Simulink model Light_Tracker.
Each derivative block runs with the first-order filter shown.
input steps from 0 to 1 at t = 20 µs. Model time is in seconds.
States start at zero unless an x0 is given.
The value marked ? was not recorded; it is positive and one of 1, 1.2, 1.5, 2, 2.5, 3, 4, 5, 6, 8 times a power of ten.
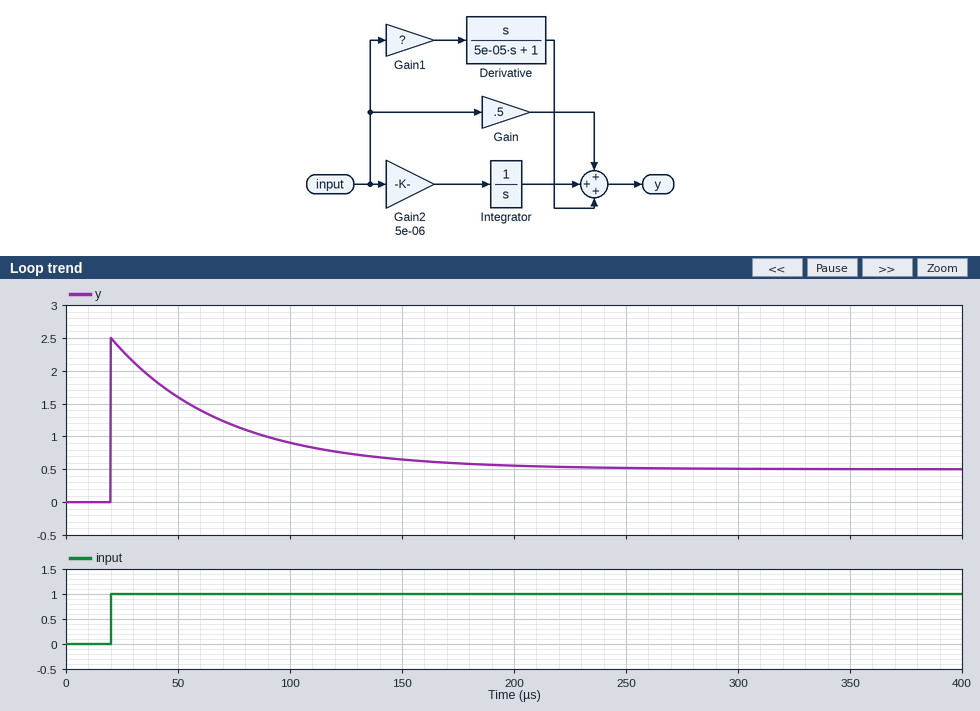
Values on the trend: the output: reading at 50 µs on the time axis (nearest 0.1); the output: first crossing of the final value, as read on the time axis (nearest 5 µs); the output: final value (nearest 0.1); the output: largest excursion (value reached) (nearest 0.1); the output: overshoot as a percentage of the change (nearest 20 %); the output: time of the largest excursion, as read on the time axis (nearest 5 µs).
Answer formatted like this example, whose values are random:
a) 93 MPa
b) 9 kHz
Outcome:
a) 1.6
b) 20 µs
c) 0.5
d) 2.5
e) 400 %
f) 20 µs
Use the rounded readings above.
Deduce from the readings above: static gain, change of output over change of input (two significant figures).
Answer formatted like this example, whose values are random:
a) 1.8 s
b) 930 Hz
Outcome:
a) 0.50
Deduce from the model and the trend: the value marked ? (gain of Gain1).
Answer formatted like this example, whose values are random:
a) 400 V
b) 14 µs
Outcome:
a) 0.0001
